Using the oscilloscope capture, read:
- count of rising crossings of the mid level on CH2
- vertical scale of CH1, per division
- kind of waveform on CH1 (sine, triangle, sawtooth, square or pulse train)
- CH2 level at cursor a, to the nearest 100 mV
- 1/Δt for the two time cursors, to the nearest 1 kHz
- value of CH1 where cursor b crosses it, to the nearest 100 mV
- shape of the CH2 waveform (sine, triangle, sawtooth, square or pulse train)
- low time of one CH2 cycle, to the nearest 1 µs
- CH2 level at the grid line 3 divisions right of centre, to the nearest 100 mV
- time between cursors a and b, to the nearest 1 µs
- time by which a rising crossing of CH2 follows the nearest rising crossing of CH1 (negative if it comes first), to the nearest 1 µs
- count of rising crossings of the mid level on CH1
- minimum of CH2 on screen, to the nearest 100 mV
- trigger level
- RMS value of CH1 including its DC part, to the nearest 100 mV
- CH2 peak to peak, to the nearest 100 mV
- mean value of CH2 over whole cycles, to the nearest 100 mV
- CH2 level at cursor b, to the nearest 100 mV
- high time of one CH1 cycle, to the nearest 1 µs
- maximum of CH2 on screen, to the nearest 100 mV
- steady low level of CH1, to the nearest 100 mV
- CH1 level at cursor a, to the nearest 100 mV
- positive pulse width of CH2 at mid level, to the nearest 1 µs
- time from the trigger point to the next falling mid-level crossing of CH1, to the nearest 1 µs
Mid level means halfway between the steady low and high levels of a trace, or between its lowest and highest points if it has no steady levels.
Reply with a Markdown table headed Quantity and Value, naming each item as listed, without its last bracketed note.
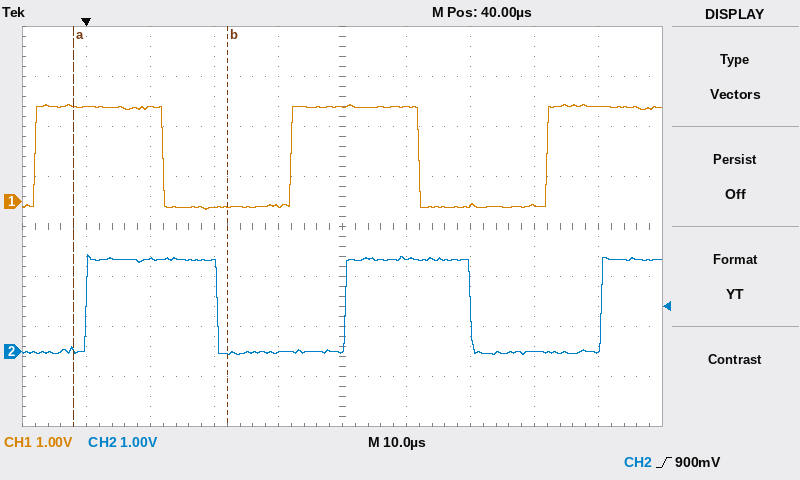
| Quantity | Value |
|---|---|
| count of rising crossings of the mid level on CH2 | 3 |
| vertical scale of CH1, per division | 1 V |
| kind of waveform on CH1 | square |
| CH2 level at cursor a, to the nearest 100 mV | 0.0 V |
| 1/Δt for the two time cursors, to the nearest 1 kHz | 42 kHz |
| value of CH1 where cursor b crosses it, to the nearest 100 mV | -100 mV |
| shape of the CH2 waveform | square |
| low time of one CH2 cycle, to the nearest 1 µs | 20 µs |
| CH2 level at the grid line 3 divisions right of centre, to the nearest 100 mV | 0.0 V |
| time between cursors a and b, to the nearest 1 µs | 24 µs |
| time by which a rising crossing of CH2 follows the nearest rising crossing of CH1 (negative if it comes first), to the nearest 1 µs | +8 µs |
| count of rising crossings of the mid level on CH1 | 3 |
| minimum of CH2 on screen, to the nearest 100 mV | -100 mV |
| trigger level | 900 mV |
| RMS value of CH1 including its DC part, to the nearest 100 mV | 1.3 V |
| CH2 peak to peak, to the nearest 100 mV | 2.0 V |
| mean value of CH2 over whole cycles, to the nearest 100 mV | 900 mV |
| CH2 level at cursor b, to the nearest 100 mV | 0.0 V |
| high time of one CH1 cycle, to the nearest 1 µs | 20 µs |
| maximum of CH2 on screen, to the nearest 100 mV | 1.9 V |
| steady low level of CH1, to the nearest 100 mV | -100 mV |
| CH1 level at cursor a, to the nearest 100 mV | 1.9 V |
| positive pulse width of CH2 at mid level, to the nearest 1 µs | 20 µs |
| time from the trigger point to the next falling mid-level crossing of CH1, to the nearest 1 µs | 12 µs |
